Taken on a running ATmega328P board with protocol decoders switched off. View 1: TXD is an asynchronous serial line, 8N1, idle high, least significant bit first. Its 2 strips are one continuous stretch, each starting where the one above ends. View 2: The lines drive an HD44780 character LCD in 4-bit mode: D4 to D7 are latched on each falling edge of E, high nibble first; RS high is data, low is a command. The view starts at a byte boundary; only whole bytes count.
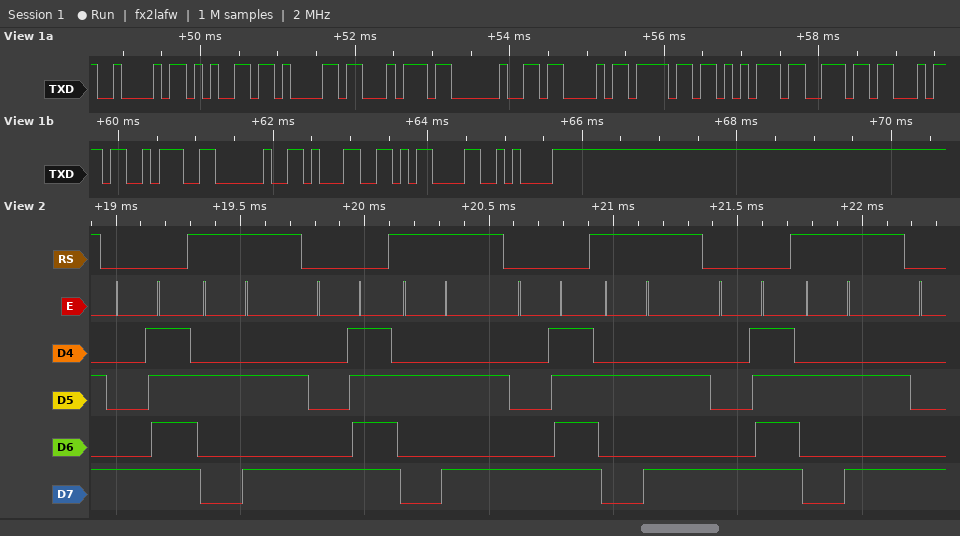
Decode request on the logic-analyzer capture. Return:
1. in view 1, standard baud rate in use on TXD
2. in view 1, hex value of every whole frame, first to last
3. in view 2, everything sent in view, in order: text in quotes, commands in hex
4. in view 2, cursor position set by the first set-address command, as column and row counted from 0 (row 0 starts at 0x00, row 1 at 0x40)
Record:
9600 baud
42 65 61 74 20 43 6F 75 6E 74 3A 20 31 0D 0A
0x8F "*" 0x8F "*" 0x8F "*" 0x8F "*"
column 15, row 0
